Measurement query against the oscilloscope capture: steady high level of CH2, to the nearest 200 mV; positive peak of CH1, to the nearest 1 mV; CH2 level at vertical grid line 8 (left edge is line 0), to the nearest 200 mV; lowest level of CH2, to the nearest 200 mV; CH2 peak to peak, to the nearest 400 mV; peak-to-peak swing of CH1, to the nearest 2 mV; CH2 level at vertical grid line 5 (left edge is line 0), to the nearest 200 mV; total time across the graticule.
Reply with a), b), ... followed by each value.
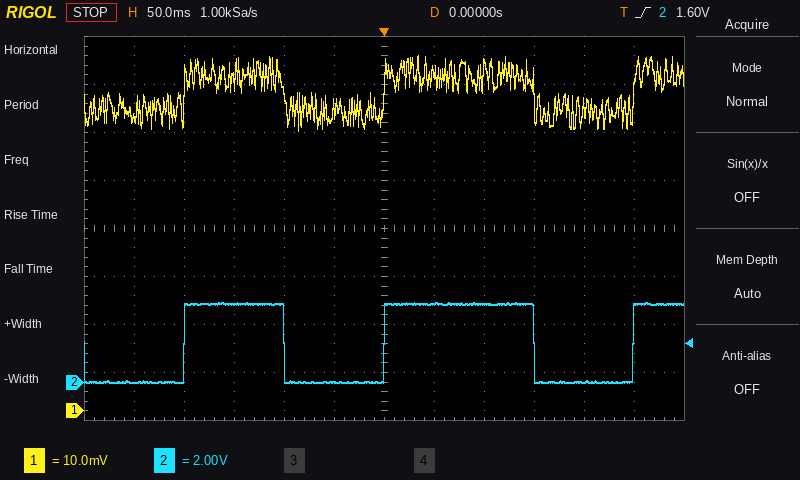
a) 3.2 V
b) 74 mV
c) 3.2 V
d) 0.0 V
e) 3.2 V
f) 16 mV
g) 0.0 V
h) 600 ms
